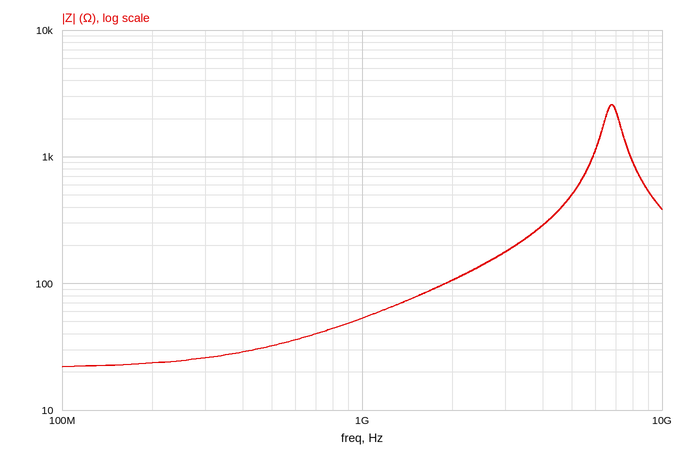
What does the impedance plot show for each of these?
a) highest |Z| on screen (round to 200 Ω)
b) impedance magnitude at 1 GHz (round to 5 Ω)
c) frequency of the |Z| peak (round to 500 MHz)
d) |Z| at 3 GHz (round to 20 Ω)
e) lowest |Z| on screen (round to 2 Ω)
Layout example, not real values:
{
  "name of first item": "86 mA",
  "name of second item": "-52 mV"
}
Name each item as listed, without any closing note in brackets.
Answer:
{
  "highest |Z| on screen": "2.6 kΩ",
  "impedance magnitude at 1 GHz": "55 Ω",
  "frequency of the |Z| peak": "7.0 GHz",
  "|Z| at 3 GHz": "180 Ω",
  "lowest |Z| on screen": "22 Ω"
}
